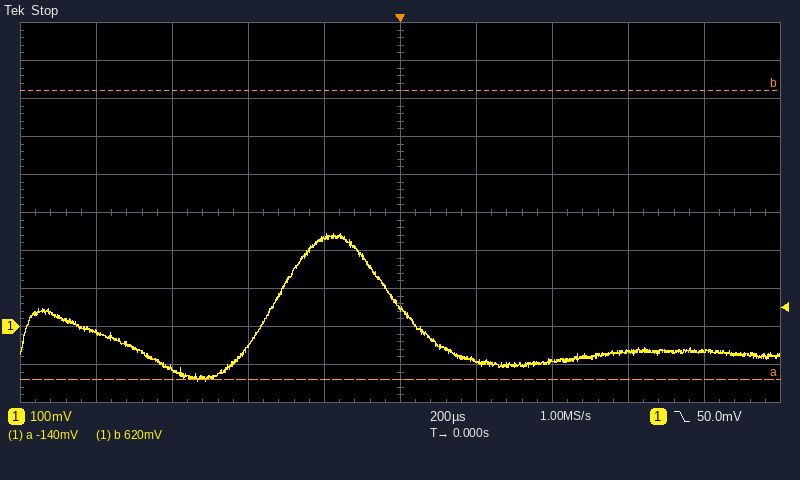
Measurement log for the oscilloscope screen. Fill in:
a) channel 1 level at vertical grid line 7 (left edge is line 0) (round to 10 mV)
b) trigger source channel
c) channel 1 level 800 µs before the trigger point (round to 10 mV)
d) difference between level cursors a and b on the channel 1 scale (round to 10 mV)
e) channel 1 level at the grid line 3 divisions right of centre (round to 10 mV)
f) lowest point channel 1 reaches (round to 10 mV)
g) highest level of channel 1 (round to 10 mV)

-90 mV
channel 1
-20 mV
760 mV
-70 mV
-140 mV
240 mV
